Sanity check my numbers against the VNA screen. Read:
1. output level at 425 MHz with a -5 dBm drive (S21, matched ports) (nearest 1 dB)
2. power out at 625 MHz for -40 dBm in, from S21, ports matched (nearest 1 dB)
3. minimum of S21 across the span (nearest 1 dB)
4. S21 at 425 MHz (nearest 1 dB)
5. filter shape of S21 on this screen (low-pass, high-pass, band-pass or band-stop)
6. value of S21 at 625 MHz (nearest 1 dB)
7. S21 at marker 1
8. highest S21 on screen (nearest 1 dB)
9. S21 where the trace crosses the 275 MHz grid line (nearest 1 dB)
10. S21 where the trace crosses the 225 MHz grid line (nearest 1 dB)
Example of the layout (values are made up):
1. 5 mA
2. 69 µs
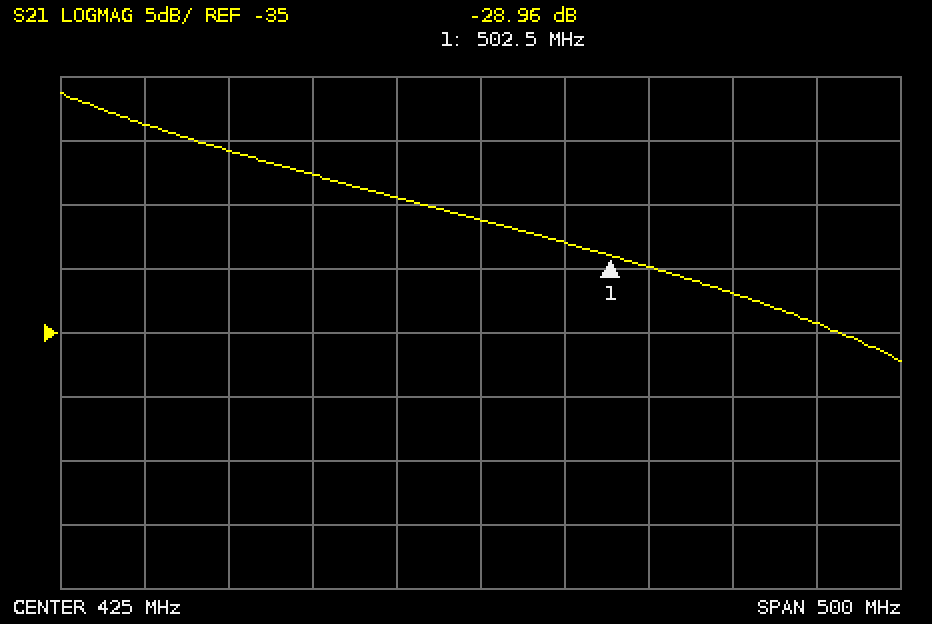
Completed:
1. -31 dBm
2. -74 dBm
3. -37 dB
4. -26 dB
5. low-pass
6. -34 dB
7. -28.96 dB
8. -16 dB
9. -21 dB
10. -19 dB
